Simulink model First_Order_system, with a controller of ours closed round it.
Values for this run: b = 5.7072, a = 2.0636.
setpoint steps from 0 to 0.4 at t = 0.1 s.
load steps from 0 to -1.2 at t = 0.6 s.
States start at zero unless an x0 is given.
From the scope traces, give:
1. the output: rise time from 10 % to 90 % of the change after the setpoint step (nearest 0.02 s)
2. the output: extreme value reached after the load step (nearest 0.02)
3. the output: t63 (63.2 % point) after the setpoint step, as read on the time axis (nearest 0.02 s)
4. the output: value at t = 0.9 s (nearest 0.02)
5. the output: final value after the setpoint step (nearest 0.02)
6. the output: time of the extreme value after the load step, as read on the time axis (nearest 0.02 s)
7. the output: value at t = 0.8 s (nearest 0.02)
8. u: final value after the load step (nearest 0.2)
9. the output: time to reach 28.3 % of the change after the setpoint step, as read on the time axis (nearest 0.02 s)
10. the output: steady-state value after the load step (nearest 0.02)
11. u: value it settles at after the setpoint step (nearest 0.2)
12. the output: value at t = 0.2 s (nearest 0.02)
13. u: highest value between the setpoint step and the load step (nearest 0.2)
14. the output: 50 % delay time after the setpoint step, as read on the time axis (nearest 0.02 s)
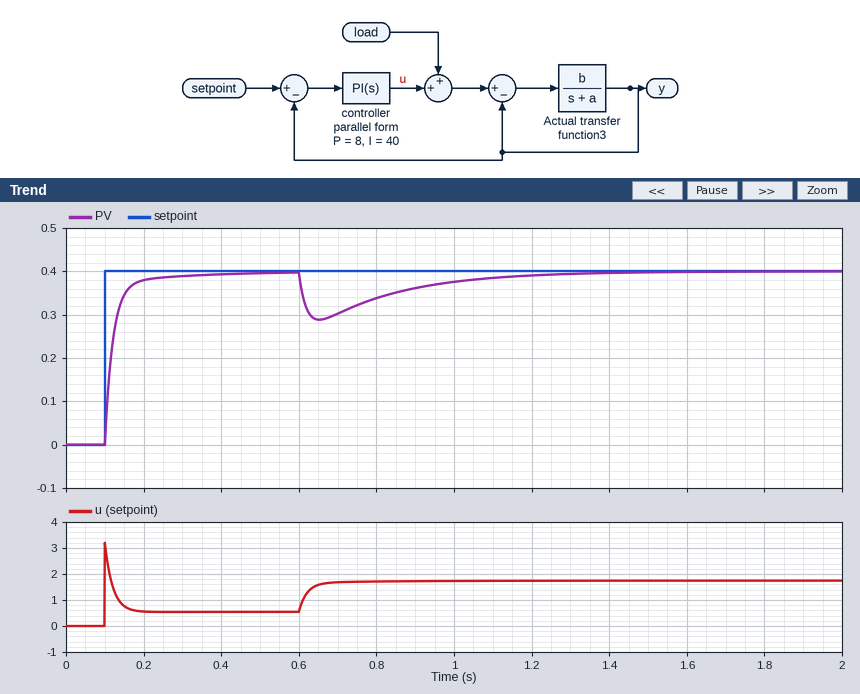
0.06 s
0.28
0.12 s
0.36
0.40
0.66 s
0.34
1.8
0.10 s
0.40
0.6
0.38
3.2
0.12 s
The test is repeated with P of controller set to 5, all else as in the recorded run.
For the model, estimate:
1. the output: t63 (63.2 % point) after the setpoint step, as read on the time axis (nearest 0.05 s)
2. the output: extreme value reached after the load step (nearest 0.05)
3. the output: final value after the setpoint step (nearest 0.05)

0.15 s
0.25
0.40
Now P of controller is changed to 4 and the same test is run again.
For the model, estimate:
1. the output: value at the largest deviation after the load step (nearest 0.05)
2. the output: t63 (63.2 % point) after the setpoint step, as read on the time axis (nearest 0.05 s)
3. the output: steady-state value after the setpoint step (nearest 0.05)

0.25
0.15 s
0.40
